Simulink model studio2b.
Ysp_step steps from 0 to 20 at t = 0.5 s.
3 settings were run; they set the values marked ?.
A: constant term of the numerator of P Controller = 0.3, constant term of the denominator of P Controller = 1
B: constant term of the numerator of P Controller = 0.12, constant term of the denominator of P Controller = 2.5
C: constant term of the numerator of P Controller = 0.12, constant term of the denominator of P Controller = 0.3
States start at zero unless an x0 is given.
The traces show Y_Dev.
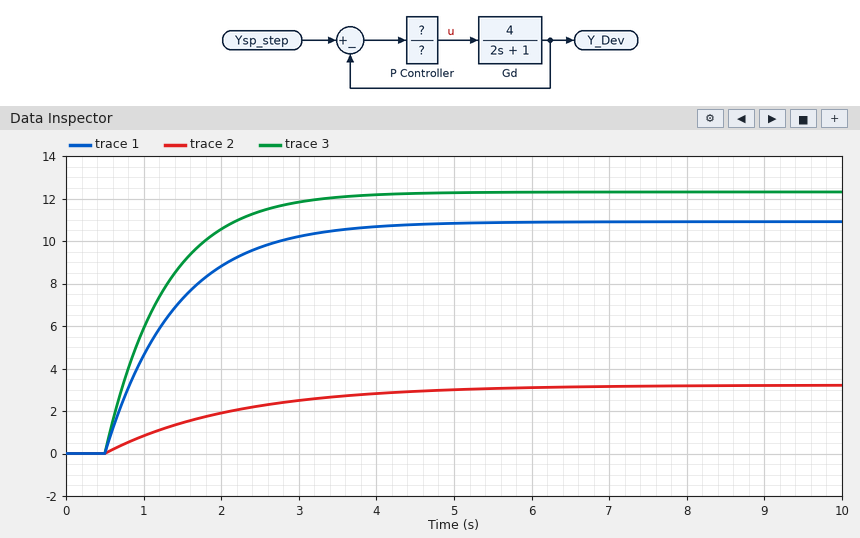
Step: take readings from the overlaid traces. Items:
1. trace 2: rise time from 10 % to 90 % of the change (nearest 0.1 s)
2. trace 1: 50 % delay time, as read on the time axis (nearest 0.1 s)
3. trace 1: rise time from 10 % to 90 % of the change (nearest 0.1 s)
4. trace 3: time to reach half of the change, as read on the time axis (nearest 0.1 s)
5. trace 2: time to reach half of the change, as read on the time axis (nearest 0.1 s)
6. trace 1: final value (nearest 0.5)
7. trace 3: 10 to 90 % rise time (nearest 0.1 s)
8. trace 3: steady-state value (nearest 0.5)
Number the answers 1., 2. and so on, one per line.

1. 3.7 s
2. 1.1 s
3. 2.0 s
4. 1.0 s
5. 1.7 s
6. 11.0
7. 1.7 s
8. 12.5
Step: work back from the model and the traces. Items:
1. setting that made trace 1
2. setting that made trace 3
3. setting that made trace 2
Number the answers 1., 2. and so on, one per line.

1. A
2. C
3. B
